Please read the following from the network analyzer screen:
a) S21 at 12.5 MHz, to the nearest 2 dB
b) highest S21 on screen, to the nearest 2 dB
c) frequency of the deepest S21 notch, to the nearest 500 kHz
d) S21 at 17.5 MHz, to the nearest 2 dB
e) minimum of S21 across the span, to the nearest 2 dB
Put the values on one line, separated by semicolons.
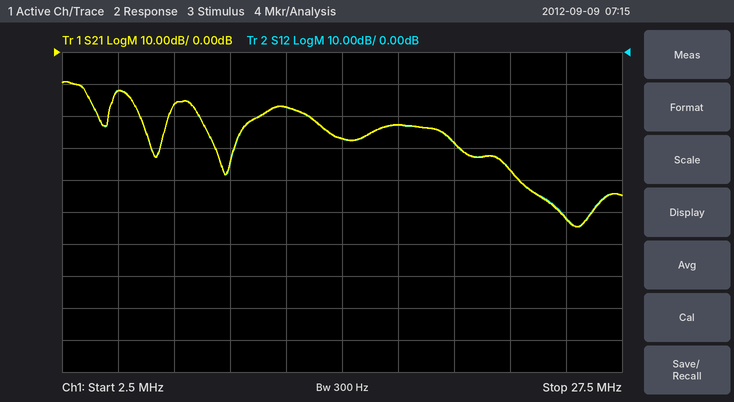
-18 dB; -10 dB; 25.5 MHz; -22 dB; -54 dB
